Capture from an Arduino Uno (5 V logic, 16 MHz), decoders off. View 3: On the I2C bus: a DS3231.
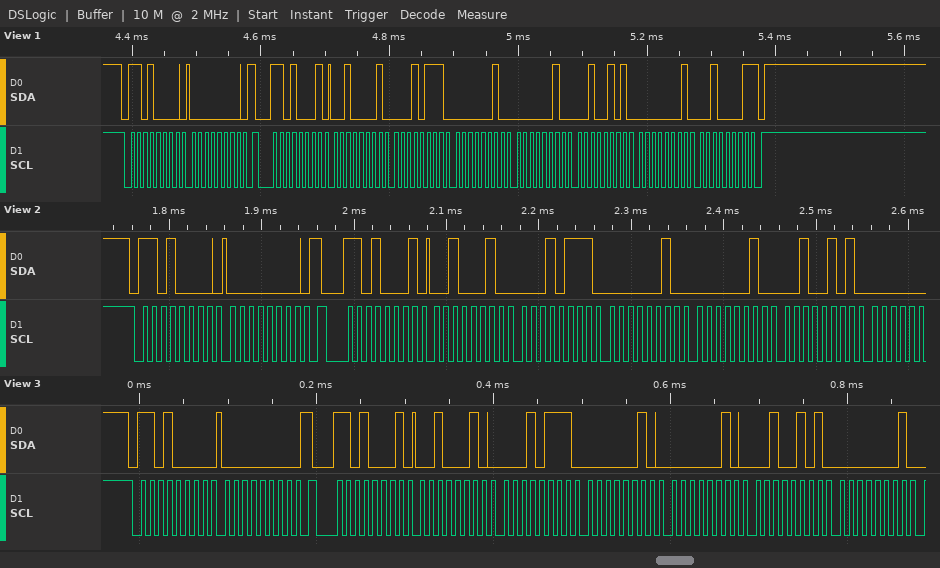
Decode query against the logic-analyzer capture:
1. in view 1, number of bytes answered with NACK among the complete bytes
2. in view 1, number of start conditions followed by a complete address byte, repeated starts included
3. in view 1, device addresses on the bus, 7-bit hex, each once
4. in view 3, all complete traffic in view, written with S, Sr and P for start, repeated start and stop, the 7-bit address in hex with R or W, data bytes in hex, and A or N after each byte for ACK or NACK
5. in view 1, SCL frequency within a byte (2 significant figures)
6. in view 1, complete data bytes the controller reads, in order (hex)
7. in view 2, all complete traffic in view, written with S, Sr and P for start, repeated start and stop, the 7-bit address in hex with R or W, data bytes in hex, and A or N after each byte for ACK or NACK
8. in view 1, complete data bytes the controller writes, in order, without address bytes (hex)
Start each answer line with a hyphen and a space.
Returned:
- 1
- 2
- 0x68
- S 68W A 00 A Sr 68R A 22 A 17 A 02 A 02 A 25 A 01 A
- 100 kHz
- 21 17 02 02 25 01 21
- S 68W A 00 A Sr 68R A 22 A 17 A 02 A 02 A 25 A
- 00
